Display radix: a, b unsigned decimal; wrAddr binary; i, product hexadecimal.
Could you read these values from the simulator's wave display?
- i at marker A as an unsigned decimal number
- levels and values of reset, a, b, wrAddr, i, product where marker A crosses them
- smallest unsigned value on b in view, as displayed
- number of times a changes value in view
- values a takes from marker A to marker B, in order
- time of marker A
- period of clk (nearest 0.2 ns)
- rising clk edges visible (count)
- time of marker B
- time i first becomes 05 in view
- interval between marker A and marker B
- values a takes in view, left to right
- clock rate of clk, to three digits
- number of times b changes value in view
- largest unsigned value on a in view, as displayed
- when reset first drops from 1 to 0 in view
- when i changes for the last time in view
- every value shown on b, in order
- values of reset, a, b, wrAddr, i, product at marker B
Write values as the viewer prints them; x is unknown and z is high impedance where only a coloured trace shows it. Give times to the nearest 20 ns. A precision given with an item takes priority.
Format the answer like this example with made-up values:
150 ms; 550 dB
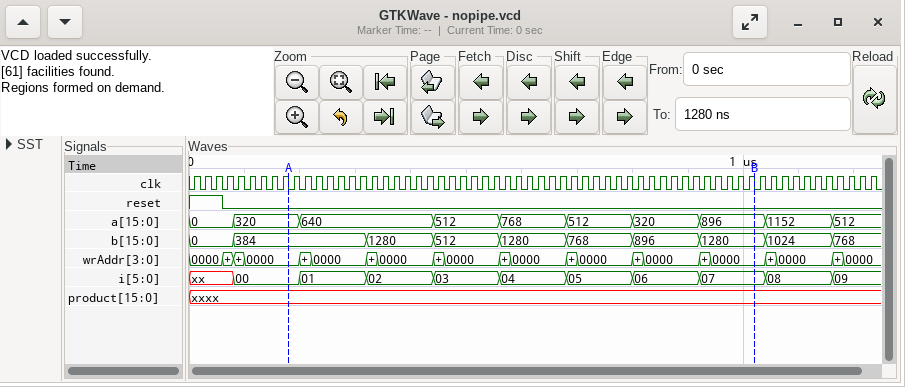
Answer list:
0; reset=0, a=320, b=384, wrAddr=0000, i=00, product=xxxx; 0; 9; 320, 640, 512, 768, 512, 320, 896; 180 ns; 20 ns; 62; 1020 ns; 680 ns; 840 ns; 0, 320, 640, 512, 768, 512, 320, 896, 1152, 512; 50.0 MHz; 9; 1152; 60 ns; 1160 ns; 0, 384, 1280, 512, 1280, 768, 896, 1280, 1024, 768; reset=0, a=896, b=1280, wrAddr=0000, i=07, product=xxxx
